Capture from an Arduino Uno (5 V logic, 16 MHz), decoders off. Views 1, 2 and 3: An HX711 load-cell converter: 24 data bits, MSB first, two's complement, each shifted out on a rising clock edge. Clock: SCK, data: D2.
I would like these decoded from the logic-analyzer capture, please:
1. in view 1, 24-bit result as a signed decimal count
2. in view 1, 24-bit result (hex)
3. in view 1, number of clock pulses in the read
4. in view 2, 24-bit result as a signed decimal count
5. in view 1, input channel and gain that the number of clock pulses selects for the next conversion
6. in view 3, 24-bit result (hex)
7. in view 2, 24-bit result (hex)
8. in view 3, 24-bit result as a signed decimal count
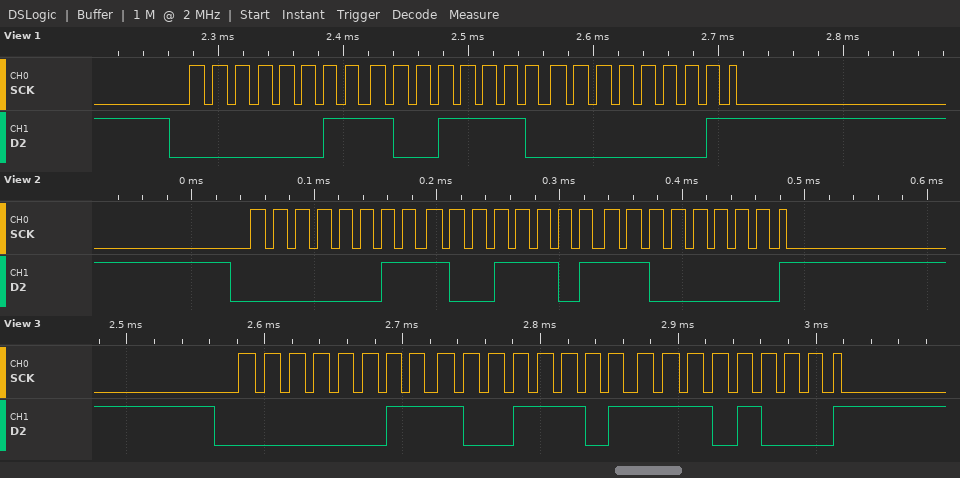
237057
0x039E01
25
236992
channel A, gain 128
0x039DE8
0x039DC0
237032
